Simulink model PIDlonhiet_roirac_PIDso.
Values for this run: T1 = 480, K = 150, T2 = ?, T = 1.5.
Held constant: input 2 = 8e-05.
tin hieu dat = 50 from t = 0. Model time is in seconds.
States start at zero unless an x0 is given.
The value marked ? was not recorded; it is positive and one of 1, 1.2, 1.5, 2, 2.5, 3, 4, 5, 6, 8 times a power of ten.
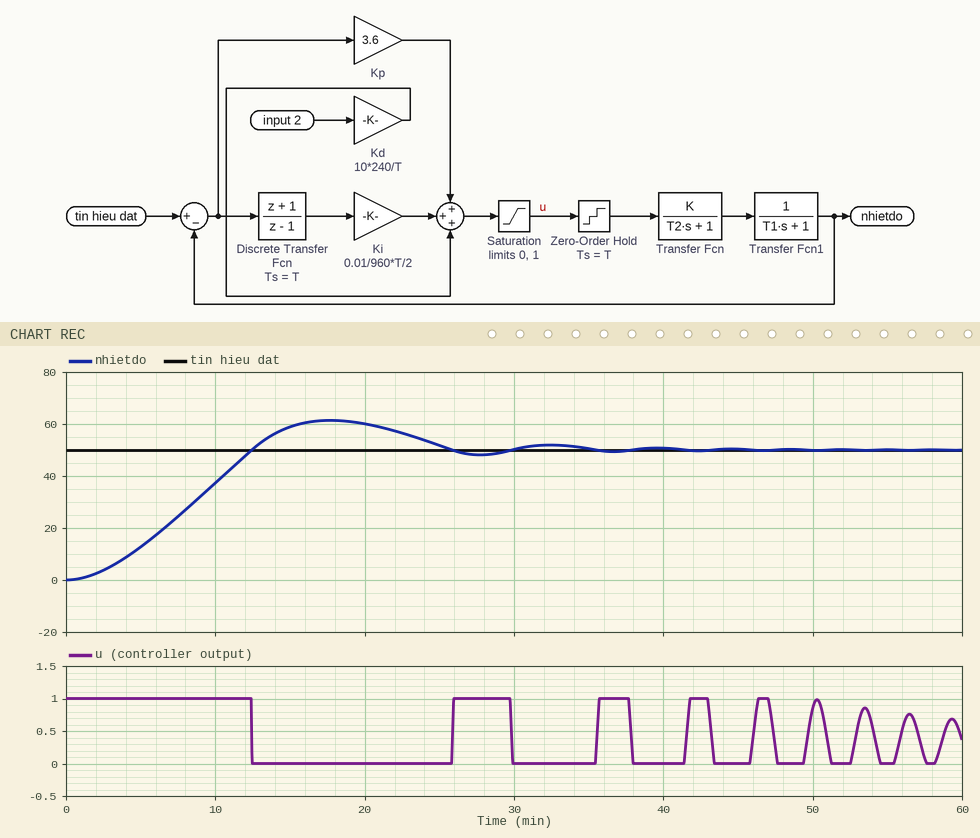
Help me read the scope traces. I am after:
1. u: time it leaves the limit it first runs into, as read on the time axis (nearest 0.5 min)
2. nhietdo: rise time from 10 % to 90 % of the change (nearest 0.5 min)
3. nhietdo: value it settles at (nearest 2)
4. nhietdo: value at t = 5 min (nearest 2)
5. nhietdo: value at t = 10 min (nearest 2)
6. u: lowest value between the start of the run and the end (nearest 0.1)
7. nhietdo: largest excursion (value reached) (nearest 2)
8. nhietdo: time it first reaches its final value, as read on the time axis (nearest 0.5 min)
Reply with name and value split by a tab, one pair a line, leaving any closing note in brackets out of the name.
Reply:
u: time it leaves the limit it first runs into, as read on the time axis	12.5 min
nhietdo: rise time from 10 % to 90 % of the change	8.5 min
nhietdo: value it settles at	50
nhietdo: value at t = 5 min	12
nhietdo: value at t = 10 min	38
u: lowest value between the start of the run and the end	0.0
nhietdo: largest excursion (value reached)	62
nhietdo: time it first reaches its final value, as read on the time axis	12.5 min
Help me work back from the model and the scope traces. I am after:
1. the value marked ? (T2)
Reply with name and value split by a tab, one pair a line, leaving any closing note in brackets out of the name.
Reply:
the value marked ?	800
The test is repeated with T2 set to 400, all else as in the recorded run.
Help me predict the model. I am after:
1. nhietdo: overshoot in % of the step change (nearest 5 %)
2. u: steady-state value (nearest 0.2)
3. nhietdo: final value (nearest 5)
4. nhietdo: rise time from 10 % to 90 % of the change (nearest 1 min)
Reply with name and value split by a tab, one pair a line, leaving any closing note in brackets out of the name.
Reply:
nhietdo: overshoot in % of the step change	25 %
u: steady-state value	0.4
nhietdo: final value	50
nhietdo: rise time from 10 % to 90 % of the change	6 min
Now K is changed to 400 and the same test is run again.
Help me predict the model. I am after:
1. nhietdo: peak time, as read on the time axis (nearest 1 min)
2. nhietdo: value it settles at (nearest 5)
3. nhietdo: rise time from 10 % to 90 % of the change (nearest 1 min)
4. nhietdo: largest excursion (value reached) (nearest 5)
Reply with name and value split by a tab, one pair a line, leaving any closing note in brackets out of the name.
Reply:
nhietdo: peak time, as read on the time axis	14 min
nhietdo: value it settles at	50
nhietdo: rise time from 10 % to 90 % of the change	4 min
nhietdo: largest excursion (value reached)	85
